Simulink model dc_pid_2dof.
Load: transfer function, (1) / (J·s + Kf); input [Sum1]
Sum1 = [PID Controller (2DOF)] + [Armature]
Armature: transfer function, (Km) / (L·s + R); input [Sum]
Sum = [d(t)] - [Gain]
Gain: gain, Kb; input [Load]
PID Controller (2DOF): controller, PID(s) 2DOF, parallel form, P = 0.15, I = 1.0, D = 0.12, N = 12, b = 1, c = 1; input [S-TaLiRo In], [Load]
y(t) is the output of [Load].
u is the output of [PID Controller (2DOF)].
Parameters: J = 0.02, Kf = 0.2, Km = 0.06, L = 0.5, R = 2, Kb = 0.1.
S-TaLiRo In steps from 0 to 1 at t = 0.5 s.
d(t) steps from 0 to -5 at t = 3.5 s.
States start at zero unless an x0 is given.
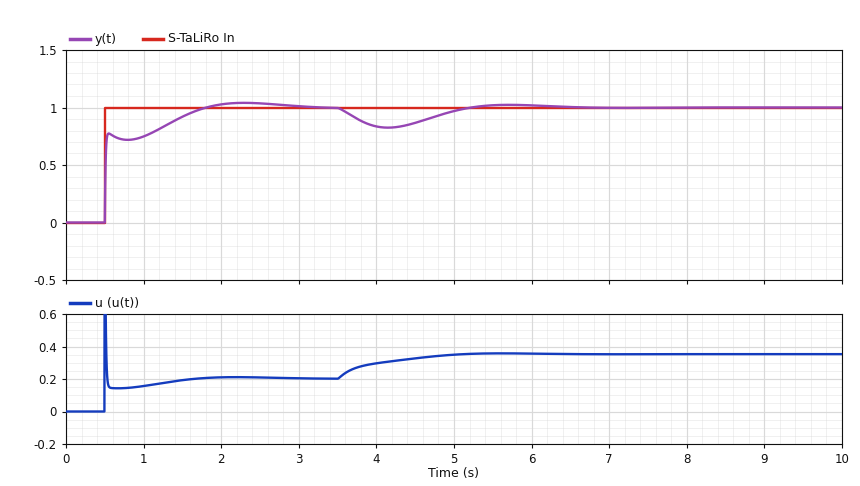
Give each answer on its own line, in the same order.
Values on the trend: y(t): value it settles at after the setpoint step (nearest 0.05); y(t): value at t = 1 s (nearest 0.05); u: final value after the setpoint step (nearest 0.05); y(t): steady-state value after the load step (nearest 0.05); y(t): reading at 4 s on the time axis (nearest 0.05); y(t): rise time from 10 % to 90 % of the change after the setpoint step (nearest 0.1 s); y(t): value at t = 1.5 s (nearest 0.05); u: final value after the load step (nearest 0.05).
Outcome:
1.00
0.75
0.20
1.00
0.85
0.9 s
0.90
0.35
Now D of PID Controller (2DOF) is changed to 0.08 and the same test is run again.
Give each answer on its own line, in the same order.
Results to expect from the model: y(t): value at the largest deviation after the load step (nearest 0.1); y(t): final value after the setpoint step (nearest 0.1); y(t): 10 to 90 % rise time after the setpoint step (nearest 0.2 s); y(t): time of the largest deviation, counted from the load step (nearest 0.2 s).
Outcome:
0.8
1.0
0.8 s
0.6 s
